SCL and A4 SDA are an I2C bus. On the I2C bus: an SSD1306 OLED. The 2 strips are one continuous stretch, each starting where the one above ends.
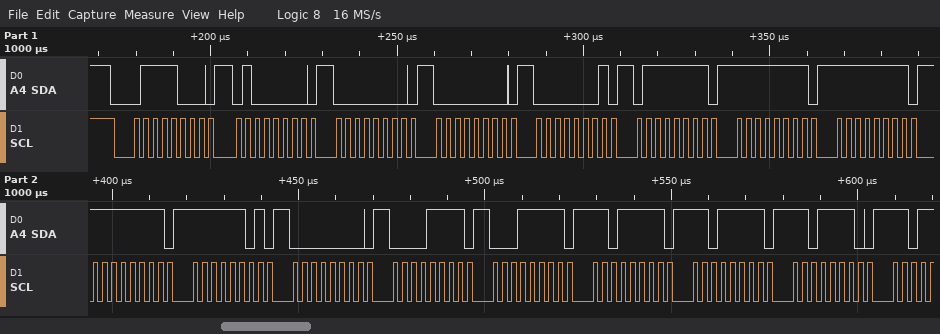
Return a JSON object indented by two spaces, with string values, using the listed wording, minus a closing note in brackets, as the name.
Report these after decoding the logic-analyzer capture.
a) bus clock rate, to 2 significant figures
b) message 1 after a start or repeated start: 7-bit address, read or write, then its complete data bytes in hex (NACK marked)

{
  "bus clock rate, to 2 significant figures": "400 kHz",
  "message 1 after a start or repeated start: 7-bit address, read or write, then its complete data bytes in hex": "0x3C write: 40 00 00 01 7F FF FF FF FD 00 0F 1F DF DF DE"
}
